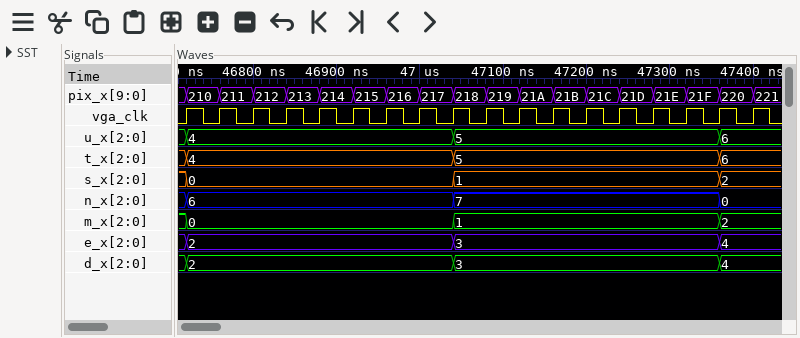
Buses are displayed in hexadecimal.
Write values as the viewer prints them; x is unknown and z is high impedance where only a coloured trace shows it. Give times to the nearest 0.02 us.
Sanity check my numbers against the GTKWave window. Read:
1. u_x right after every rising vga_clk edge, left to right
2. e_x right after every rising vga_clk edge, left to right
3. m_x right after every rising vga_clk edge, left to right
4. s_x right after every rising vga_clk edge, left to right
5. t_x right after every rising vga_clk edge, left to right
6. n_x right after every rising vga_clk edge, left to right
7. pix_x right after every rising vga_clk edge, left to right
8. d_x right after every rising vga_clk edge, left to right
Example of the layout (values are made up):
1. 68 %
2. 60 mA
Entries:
1. 4, 4, 4, 4, 4, 4, 4, 4, 5, 5, 5, 5, 5, 5, 5, 5, 6, 6
2. 2, 2, 2, 2, 2, 2, 2, 2, 3, 3, 3, 3, 3, 3, 3, 3, 4, 4
3. 0, 0, 0, 0, 0, 0, 0, 0, 1, 1, 1, 1, 1, 1, 1, 1, 2, 2
4. 0, 0, 0, 0, 0, 0, 0, 0, 1, 1, 1, 1, 1, 1, 1, 1, 2, 2
5. 4, 4, 4, 4, 4, 4, 4, 4, 5, 5, 5, 5, 5, 5, 5, 5, 6, 6
6. 6, 6, 6, 6, 6, 6, 6, 6, 7, 7, 7, 7, 7, 7, 7, 7, 0, 0
7. 210, 211, 212, 213, 214, 215, 216, 217, 218, 219, 21A, 21B, 21C, 21D, 21E, 21F, 220, 221
8. 2, 2, 2, 2, 2, 2, 2, 2, 3, 3, 3, 3, 3, 3, 3, 3, 4, 4
